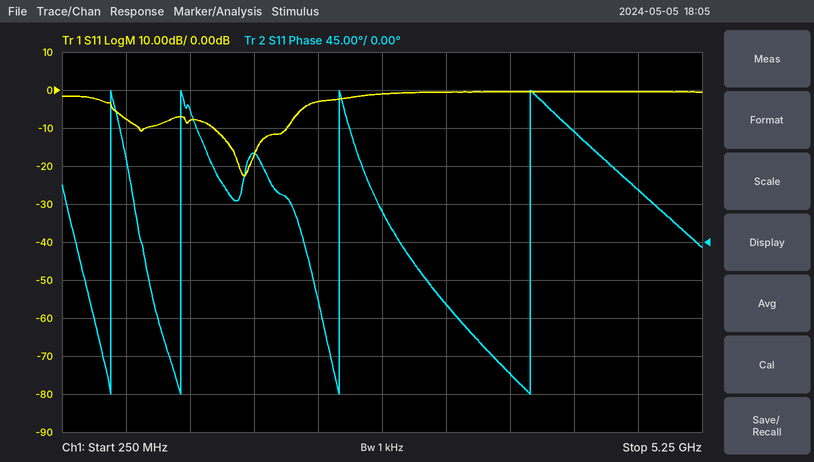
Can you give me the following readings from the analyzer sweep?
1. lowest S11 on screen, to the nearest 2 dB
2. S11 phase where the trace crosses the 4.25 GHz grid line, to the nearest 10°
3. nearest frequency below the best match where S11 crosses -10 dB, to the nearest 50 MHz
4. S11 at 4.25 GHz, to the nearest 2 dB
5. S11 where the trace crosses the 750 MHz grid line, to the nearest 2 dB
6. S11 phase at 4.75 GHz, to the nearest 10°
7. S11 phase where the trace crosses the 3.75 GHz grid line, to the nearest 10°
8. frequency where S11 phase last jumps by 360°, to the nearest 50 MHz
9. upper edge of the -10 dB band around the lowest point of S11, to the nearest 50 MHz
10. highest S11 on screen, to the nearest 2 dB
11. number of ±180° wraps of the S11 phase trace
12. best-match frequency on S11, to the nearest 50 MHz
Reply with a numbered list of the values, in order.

1. -22 dB
2. 130°
3. 1.45 GHz
4. 0 dB
5. -8 dB
6. 60°
7. -160°
8. 3.90 GHz
9. 2.00 GHz
10. 0 dB
11. 4
12. 1.65 GHz
